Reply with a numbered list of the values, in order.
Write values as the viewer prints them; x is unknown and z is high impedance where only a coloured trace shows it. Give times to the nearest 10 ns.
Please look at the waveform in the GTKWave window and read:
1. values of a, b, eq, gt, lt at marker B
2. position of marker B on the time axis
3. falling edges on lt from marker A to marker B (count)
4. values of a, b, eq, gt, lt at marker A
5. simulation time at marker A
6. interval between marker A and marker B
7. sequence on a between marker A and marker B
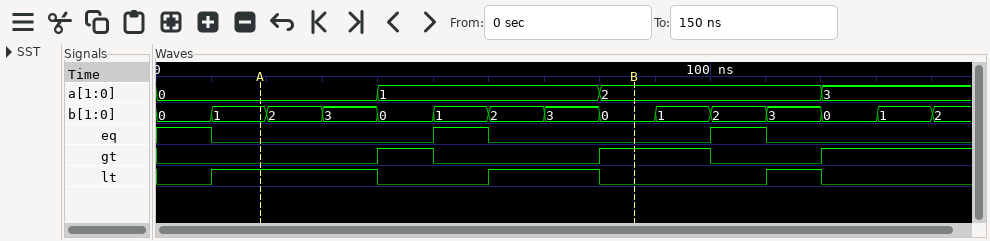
1. a=2, b=0, eq=0, gt=1, lt=0
2. 90 ns
3. 2
4. a=0, b=1, eq=0, gt=0, lt=1
5. 20 ns
6. 70 ns
7. 0, 1, 2
